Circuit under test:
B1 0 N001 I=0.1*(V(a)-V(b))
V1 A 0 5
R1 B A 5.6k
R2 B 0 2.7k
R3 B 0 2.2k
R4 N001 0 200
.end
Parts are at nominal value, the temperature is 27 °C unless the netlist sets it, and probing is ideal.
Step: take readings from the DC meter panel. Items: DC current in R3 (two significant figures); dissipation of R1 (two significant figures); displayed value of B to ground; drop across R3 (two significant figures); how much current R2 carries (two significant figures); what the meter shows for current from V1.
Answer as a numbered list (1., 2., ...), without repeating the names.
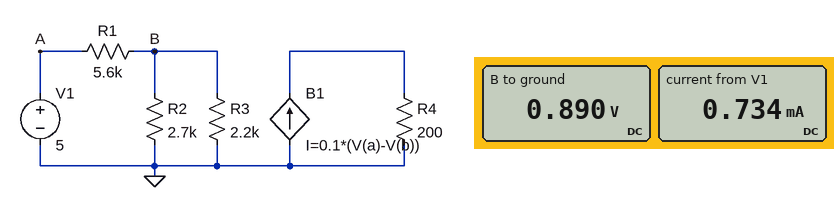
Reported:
1. 400 µA
2. 3.0 mW
3. 0.890 V
4. 890 mV
5. 330 µA
6. 0.734 mA
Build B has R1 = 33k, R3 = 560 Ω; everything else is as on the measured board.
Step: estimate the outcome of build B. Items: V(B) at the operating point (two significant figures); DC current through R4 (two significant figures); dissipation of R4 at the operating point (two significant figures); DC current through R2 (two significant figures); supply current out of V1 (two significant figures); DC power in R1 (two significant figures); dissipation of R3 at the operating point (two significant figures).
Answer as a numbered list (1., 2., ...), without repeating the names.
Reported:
1. 69 mV
2. 490 mA
3. 49 W
4. 26 µA
5. 150 µA
6. 740 µW
7. 8.6 µW
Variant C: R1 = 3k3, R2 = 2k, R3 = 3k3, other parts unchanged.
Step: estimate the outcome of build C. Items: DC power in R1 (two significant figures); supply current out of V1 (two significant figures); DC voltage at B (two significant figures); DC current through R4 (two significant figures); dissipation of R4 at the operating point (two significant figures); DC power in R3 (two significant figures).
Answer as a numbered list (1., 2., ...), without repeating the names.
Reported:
1. 4.0 mW
2. 1.1 mA
3. 1.4 V
4. 360 mA
5. 26 W
6. 570 µW
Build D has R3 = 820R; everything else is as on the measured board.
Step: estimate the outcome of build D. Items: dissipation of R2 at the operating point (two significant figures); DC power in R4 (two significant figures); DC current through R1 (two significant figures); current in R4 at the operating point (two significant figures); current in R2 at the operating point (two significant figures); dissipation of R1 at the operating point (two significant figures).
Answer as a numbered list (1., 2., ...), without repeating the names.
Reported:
1. 94 µW
2. 40 W
3. 800 µA
4. 450 mA
5. 190 µA
6. 3.6 mW
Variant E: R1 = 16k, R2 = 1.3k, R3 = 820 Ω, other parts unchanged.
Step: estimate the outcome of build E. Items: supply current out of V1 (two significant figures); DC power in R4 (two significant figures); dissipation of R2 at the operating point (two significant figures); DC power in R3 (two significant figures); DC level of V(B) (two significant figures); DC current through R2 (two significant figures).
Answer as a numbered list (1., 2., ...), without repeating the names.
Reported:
1. 300 µA
2. 47 W
3. 18 µW
4. 28 µW
5. 150 mV
6. 120 µA
